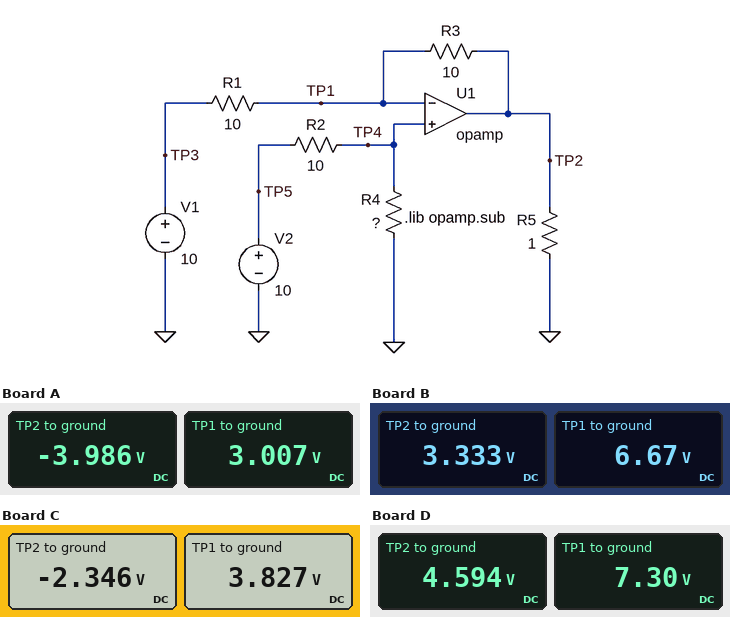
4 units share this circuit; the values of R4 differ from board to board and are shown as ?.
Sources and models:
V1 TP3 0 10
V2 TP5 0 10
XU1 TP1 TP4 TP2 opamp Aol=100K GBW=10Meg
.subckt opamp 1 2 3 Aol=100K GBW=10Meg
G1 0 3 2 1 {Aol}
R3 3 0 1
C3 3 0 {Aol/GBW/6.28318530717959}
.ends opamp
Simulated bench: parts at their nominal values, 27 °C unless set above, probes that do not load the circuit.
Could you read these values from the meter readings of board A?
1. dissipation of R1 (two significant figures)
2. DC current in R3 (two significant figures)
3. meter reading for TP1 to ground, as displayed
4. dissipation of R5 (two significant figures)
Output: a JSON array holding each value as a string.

["4.9 W", "700 mA", "3.007 V", "16 W"]
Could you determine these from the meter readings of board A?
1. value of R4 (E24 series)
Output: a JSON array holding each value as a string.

["4.3 Ω"]
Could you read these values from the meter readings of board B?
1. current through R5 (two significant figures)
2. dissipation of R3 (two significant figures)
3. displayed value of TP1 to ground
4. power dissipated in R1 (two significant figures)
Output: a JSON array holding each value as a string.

["3.3 A", "1.1 W", "6.67 V", "1.1 W"]
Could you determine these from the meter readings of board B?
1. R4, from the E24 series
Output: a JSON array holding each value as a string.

["20 Ω"]
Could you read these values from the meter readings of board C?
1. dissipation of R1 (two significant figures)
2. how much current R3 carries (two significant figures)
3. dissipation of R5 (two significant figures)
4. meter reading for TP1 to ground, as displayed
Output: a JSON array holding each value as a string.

["3.8 W", "620 mA", "5.5 W", "3.827 V"]
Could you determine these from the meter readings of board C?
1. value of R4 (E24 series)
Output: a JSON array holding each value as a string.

["6.2 Ω"]
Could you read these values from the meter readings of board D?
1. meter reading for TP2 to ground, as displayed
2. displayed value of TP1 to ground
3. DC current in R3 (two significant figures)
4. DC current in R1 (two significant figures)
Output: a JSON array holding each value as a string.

["4.594 V", "7.30 V", "270 mA", "270 mA"]
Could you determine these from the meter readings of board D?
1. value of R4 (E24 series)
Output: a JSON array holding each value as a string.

["27 Ω"]
